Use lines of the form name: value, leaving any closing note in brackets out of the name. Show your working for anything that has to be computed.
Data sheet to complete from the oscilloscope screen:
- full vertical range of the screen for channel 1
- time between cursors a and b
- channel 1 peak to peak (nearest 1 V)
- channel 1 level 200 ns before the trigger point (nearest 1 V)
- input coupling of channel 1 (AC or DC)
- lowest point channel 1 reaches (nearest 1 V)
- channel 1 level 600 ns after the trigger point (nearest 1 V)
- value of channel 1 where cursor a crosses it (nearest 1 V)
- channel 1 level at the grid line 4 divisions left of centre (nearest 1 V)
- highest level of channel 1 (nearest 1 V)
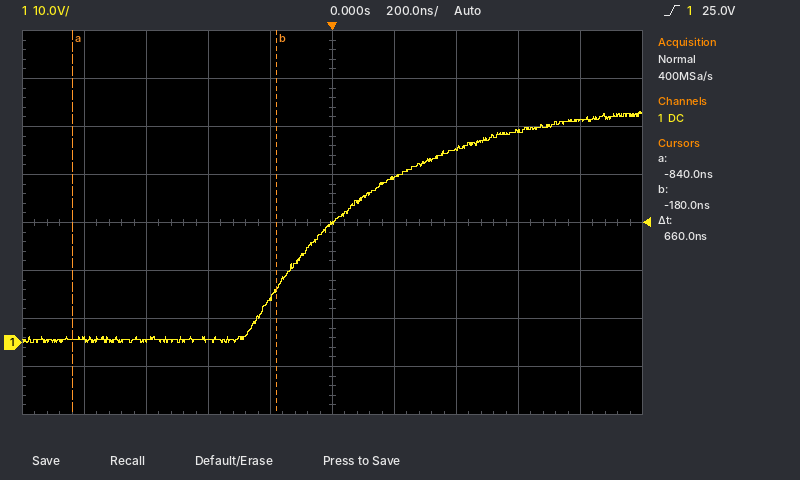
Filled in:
full vertical range of the screen for channel 1: 80 V
time between cursors a and b: 660 ns
channel 1 peak to peak: 48 V − (0 V) = 48 V
channel 1 level 200 ns before the trigger point: 9 V
input coupling of channel 1: DC
lowest point channel 1 reaches: 0 V
channel 1 level 600 ns after the trigger point: 44 V
value of channel 1 where cursor a crosses it: 1 V
channel 1 level at the grid line 4 divisions left of centre: 1 V
highest level of channel 1: 48 V
